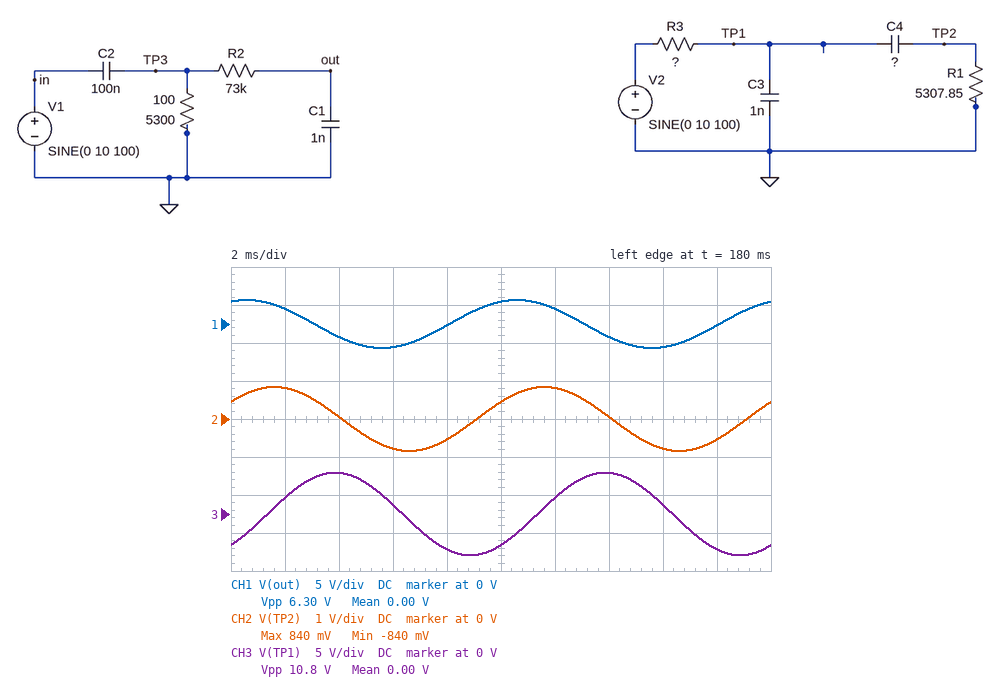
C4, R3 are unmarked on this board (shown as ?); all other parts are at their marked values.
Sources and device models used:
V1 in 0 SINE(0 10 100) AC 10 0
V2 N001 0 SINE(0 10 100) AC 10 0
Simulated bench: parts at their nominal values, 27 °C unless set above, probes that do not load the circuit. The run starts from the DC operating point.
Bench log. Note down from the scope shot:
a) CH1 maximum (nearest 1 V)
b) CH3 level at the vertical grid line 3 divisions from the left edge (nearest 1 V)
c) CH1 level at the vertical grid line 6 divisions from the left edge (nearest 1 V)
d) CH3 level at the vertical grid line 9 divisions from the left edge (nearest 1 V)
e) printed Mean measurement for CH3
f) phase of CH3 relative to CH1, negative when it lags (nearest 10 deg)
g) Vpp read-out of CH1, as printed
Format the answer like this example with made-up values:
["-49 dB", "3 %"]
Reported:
["3 V", "1 V", "2 V", "-5 V", "0.00 V", "-120 deg", "6.30 V"]
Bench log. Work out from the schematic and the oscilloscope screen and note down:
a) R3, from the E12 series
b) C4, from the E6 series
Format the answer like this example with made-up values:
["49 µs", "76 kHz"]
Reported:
["47 kΩ", "47 nF"]
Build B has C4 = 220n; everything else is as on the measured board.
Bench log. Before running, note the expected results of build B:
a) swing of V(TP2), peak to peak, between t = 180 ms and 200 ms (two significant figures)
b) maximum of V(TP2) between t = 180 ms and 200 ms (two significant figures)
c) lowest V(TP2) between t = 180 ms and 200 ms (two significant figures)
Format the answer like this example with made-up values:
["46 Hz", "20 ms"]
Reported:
["2.0 V", "1.0 V", "-1.0 V"]
